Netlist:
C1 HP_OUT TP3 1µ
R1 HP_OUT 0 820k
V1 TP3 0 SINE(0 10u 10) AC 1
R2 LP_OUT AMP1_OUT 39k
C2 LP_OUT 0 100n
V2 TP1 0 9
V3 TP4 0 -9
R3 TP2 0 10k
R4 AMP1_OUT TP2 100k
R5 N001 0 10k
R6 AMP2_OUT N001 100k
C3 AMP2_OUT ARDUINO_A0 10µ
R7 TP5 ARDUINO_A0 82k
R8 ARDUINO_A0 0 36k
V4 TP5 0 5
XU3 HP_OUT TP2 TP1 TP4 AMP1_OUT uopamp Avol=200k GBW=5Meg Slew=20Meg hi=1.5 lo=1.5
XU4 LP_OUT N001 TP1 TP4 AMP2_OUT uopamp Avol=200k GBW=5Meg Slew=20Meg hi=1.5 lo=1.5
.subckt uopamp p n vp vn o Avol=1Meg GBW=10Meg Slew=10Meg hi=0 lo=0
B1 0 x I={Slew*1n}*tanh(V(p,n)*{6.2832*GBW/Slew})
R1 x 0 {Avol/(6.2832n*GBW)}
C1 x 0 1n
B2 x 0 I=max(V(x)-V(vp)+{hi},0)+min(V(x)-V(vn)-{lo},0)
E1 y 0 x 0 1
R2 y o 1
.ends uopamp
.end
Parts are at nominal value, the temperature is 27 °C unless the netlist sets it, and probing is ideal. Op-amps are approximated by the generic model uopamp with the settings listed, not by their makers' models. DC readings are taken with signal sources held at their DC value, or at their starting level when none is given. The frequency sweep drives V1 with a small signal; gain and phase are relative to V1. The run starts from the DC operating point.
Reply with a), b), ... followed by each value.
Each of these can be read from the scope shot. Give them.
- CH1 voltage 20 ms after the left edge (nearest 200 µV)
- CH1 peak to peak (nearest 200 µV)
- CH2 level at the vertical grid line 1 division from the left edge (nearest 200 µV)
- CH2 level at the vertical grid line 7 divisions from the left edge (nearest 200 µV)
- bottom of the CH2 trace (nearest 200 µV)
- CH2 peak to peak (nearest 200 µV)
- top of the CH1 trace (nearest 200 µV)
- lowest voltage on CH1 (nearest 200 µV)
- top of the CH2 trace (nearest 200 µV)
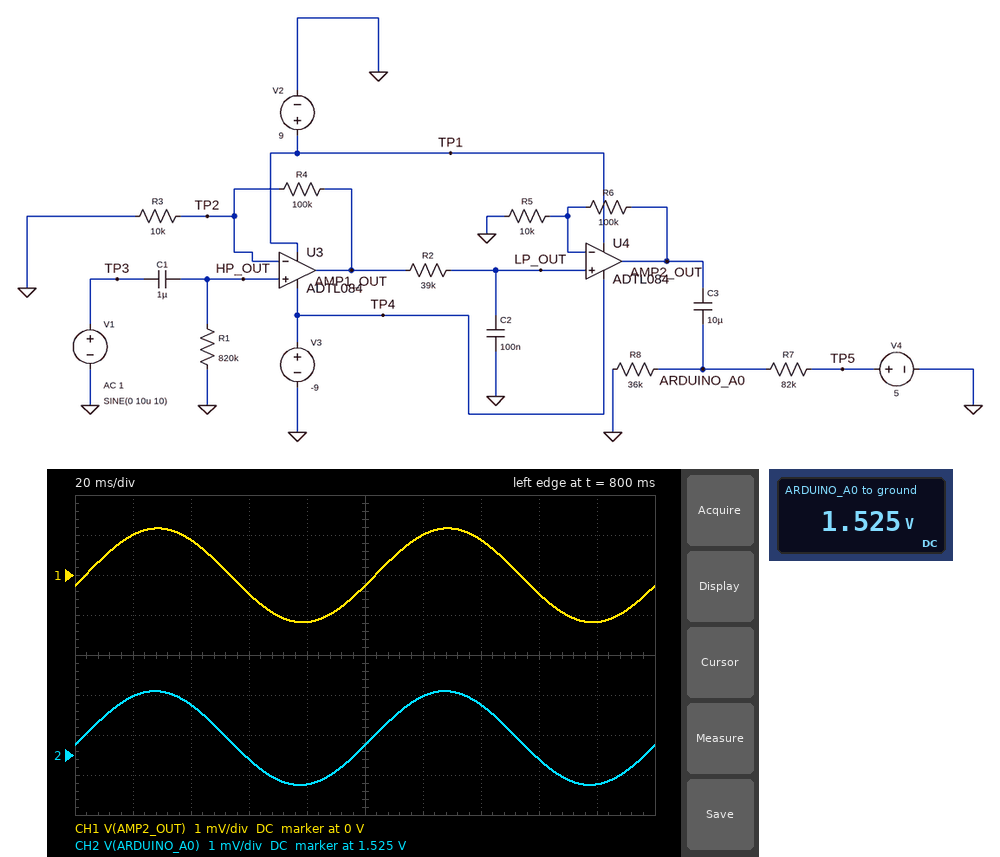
a) 1.0 mV
b) 2.4 mV
c) 1.5264 V
d) 1.5262 V
e) 1.5242 V
f) 2.4 mV
g) 1.2 mV
h) -1.2 mV
i) 1.5266 V
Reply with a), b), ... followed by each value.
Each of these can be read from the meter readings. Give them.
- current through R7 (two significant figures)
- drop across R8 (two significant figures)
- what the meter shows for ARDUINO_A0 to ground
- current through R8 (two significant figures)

a) 42 µA
b) 1.5 V
c) 1.525 V
d) 42 µA
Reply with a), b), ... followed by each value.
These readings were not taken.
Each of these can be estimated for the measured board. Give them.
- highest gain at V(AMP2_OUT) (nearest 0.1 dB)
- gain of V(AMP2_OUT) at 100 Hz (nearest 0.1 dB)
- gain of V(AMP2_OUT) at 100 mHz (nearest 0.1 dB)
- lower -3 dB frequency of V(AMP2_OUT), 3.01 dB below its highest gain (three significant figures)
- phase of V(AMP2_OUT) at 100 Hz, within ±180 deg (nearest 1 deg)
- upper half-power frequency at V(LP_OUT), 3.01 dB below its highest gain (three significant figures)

a) 41.6 dB
b) 33.2 dB
c) 34.9 dB
d) 192 mHz
e) -68 deg
f) 41.2 Hz
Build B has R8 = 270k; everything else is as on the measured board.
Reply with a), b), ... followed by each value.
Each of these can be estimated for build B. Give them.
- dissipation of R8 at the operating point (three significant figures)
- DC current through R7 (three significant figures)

a) 54.5 µW
b) 14.2 µA
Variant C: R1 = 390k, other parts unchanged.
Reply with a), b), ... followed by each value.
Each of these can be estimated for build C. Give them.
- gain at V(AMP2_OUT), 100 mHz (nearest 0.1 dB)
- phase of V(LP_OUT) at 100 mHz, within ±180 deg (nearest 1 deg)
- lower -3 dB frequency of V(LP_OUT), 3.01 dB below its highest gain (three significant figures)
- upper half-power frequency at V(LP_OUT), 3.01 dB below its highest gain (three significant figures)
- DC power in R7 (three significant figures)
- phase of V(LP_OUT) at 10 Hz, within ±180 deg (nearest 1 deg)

a) 29.2 dB
b) 76 deg
c) 400 mHz
d) 41.6 Hz
e) 147 µW
f) -11 deg
